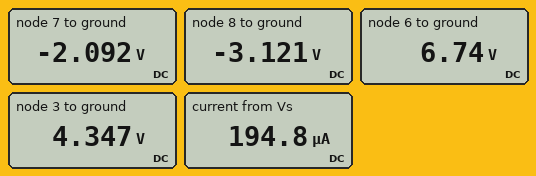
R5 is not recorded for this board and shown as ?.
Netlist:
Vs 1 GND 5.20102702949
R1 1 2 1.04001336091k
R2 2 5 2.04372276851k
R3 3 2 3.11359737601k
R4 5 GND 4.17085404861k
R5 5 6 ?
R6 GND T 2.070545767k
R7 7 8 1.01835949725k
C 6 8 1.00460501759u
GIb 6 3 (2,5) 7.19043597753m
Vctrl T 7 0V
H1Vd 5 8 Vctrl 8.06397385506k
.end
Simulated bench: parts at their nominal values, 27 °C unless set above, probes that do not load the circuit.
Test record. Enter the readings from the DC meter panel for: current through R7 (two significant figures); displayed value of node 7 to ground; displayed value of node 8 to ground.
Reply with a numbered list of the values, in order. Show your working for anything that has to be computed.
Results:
1. (-2.092 V - (-3.121 V)) / 1.018 kΩ = 1.0 mA
2. -2.092 V
3. -3.121 V
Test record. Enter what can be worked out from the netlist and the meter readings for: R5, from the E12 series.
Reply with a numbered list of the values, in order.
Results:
1. 8.2 kΩ
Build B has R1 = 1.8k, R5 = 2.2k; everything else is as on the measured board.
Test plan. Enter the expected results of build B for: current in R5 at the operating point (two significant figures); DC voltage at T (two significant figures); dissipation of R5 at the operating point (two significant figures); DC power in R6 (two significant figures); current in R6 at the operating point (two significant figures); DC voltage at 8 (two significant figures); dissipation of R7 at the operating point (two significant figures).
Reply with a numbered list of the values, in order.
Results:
1. 200 µA
2. -2.0 V
3. 91 µW
4. 2.0 mW
5. 980 µA
6. -3.0 V
7. 980 µW
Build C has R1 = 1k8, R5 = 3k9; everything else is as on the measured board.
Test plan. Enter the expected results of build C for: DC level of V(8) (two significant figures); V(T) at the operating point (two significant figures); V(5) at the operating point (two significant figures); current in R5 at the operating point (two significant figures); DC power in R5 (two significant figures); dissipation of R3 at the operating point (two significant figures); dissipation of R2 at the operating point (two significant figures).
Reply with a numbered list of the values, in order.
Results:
1. -3.0 V
2. -2.0 V
3. 4.9 V
4. 200 µA
5. 160 µW
6. 130 µW
7. 390 nW
